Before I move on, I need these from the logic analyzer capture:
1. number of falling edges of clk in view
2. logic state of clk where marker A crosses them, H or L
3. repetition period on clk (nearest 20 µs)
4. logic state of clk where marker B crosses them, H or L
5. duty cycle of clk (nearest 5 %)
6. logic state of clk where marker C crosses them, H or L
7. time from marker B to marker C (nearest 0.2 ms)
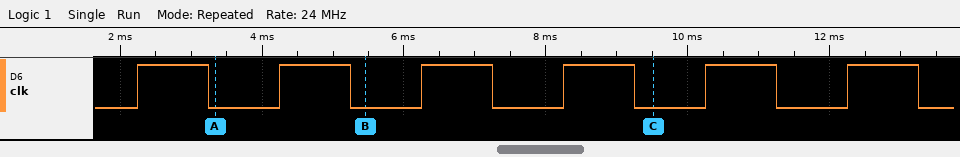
6
clk=L
2000 µs
clk=L
50 %
clk=L
4 ms
